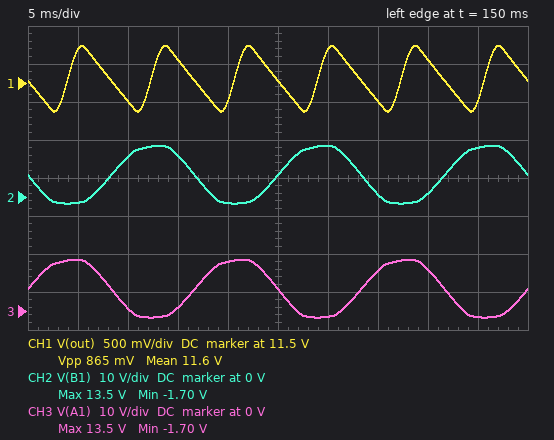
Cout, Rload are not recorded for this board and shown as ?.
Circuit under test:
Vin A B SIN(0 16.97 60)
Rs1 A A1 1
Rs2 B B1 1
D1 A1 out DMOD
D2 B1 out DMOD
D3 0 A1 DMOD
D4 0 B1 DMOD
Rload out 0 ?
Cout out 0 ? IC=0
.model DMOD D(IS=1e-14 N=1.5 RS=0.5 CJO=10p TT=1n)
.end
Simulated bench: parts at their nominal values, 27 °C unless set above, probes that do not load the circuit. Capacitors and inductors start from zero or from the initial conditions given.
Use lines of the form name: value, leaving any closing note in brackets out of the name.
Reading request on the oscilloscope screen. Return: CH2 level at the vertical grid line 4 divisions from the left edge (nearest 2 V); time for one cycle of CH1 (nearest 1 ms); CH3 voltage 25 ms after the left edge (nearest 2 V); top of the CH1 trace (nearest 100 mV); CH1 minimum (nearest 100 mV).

CH2 level at the vertical grid line 4 divisions from the left edge: -2 V
time for one cycle of CH1: 8 ms
CH3 voltage 25 ms after the left edge: 6 V
top of the CH1 trace: 12.0 V
CH1 minimum: 11.1 V
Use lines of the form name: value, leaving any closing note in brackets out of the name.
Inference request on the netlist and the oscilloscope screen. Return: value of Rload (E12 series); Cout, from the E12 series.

value of Rload: 47 Ω
Cout, from the E12 series: 1.5 mF
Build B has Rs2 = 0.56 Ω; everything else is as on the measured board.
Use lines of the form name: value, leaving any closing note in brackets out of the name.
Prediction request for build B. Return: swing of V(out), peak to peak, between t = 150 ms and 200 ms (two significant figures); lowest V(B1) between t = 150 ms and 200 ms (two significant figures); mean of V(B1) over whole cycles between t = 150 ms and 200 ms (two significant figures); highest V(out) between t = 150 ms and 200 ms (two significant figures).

swing of V(out), peak to peak, between t = 150 ms and 200 ms: 910 mV
lowest V(B1) between t = 150 ms and 200 ms: -1.8 V
mean of V(B1) over whole cycles between t = 150 ms and 200 ms: 5.9 V
highest V(out) between t = 150 ms and 200 ms: 12 V
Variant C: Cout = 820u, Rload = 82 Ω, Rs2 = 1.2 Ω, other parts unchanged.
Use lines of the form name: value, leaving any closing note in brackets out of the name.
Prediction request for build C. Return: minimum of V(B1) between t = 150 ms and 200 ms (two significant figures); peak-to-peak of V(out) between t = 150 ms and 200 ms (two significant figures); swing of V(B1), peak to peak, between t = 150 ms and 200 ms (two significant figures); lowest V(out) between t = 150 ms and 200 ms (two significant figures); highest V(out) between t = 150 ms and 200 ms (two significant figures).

minimum of V(B1) between t = 150 ms and 200 ms: -1.6 V
peak-to-peak of V(out) between t = 150 ms and 200 ms: 1.0 V
swing of V(B1), peak to peak, between t = 150 ms and 200 ms: 16 V
lowest V(out) between t = 150 ms and 200 ms: 12 V
highest V(out) between t = 150 ms and 200 ms: 13 V
